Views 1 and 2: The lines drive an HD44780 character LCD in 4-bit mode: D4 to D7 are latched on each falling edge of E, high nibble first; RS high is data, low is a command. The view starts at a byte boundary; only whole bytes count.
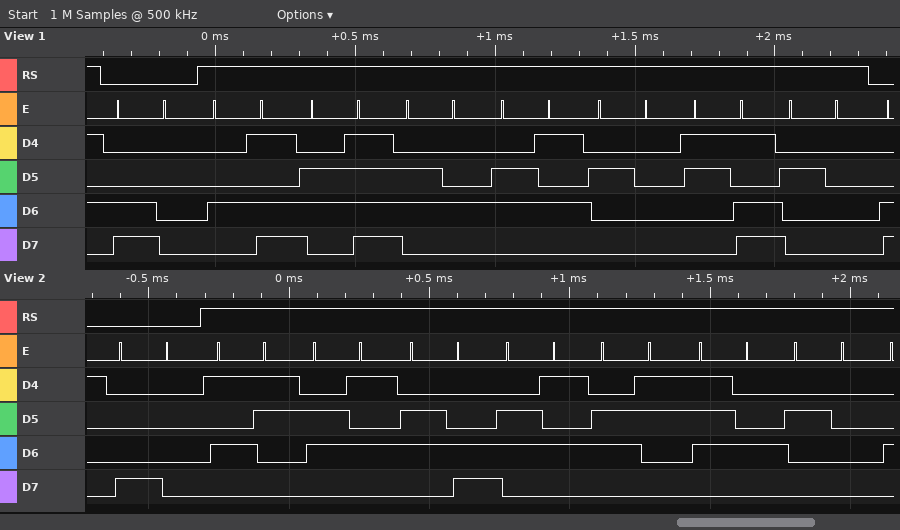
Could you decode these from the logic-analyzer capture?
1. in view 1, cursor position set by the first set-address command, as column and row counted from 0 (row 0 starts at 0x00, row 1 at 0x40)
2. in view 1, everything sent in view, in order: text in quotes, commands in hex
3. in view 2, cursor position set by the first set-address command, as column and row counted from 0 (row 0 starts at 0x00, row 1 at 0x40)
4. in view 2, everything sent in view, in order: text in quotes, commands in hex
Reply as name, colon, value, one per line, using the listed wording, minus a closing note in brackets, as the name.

in view 1, cursor position set by the first set-address command, as column and row counted from 0: column 0, row 1
in view 1, everything sent in view, in order: text in quotes, commands in hex: 0xC0 "Mode = "
in view 2, cursor position set by the first set-address command, as column and row counted from 0: column 0, row 0
in view 2, everything sent in view, in order: text in quotes, commands in hex: 0x80 "Select "
